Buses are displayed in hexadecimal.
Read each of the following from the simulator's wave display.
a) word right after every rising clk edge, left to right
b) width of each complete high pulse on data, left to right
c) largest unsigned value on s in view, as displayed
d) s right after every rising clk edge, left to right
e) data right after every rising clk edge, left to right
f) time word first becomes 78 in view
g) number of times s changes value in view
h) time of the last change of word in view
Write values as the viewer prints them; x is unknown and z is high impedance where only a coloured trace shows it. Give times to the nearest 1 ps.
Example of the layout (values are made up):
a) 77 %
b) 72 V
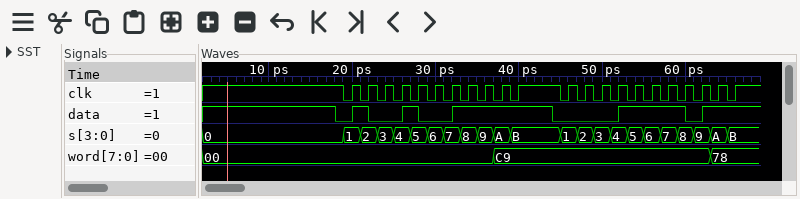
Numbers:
a) 00, 00, 00, 00, 00, 00, 00, 00, 00, C9, C9, C9, C9, C9, C9, C9, C9, C9, C9, C9, 78, 78
b) 2 ps, 2 ps, 12 ps, 8 ps
c) B
d) 1, 2, 3, 4, 5, 6, 7, 8, 9, A, B, 1, 2, 3, 4, 5, 6, 7, 8, 9, A, B
e) 1 0 0 1 0 0 1 1 1 1 1 0 0 0 1 1 1 1 0 1 1 1
f) 63 ps
g) 22
h) 63 ps
